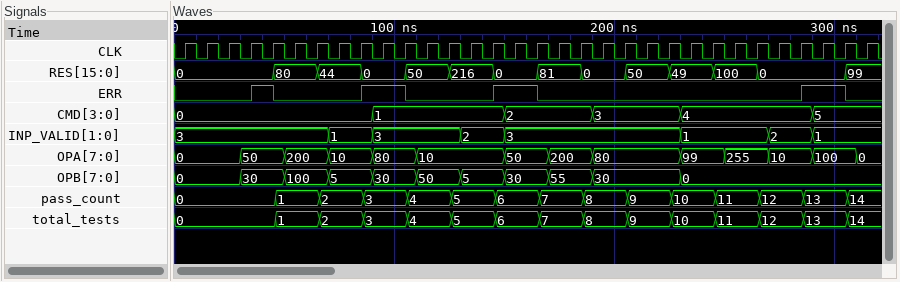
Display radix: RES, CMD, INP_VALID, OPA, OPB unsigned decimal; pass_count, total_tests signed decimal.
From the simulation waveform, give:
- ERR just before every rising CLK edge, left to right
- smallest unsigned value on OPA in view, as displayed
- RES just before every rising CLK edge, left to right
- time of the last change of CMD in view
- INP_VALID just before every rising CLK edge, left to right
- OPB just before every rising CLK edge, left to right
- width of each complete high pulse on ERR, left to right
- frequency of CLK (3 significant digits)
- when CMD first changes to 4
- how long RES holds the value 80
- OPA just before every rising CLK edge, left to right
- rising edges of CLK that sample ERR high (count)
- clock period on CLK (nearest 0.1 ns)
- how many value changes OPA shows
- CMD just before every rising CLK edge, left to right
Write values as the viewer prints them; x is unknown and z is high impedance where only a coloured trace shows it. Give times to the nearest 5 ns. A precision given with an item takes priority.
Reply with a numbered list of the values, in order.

1. 0 0 0 0 1 0 0 0 0 1 1 0 0 0 0 1 1 0 0 0 0 0 0 0 0 0 0 0 0 1 1 0
2. 0
3. 0, 0, 0, 0, 0, 80, 80, 44, 44, 0, 0, 50, 50, 216, 216, 0, 0, 81, 81, 0, 0, 50, 50, 49, 49, 100, 100, 0, 0, 0, 0, 99
4. 290 ns
5. 3, 3, 3, 3, 3, 3, 3, 1, 1, 3, 3, 3, 3, 2, 2, 3, 3, 3, 3, 3, 3, 3, 3, 1, 1, 1, 1, 2, 2, 1, 1, 1
6. 0, 0, 0, 30, 30, 100, 100, 5, 5, 30, 30, 50, 50, 5, 5, 30, 30, 55, 55, 30, 30, 30, 30, 0, 0, 0, 0, 0, 0, 0, 0, 0
7. 10 ns, 20 ns, 20 ns, 20 ns
8. 100 MHz
9. 230 ns
10. 20 ns
11. 0, 0, 0, 50, 50, 200, 200, 10, 10, 80, 80, 10, 10, 10, 10, 50, 50, 200, 200, 80, 80, 80, 80, 99, 99, 255, 255, 10, 10, 100, 100, 0
12. 7
13. 10 ns
14. 13
15. 0, 0, 0, 0, 0, 0, 0, 0, 0, 1, 1, 1, 1, 1, 1, 2, 2, 2, 2, 3, 3, 3, 3, 4, 4, 4, 4, 4, 4, 5, 5, 5
